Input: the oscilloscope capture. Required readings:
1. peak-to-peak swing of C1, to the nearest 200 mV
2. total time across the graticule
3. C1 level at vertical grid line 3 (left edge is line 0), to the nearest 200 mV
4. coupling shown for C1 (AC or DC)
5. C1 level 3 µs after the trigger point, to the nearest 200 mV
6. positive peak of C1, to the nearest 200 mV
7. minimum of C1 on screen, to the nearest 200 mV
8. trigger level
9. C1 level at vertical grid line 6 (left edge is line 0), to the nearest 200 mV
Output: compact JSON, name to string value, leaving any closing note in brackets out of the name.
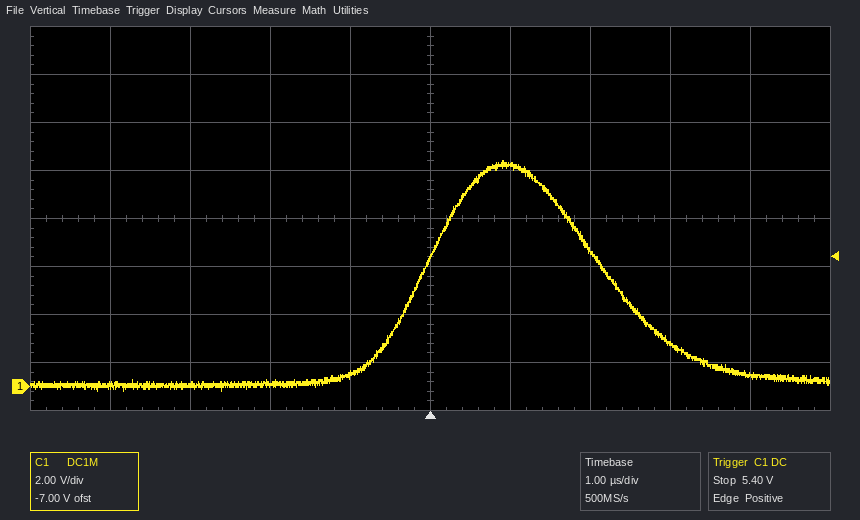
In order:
{"peak-to-peak swing of C1, to the nearest 200 mV": "9.6 V", "total time across the graticule": "10 µs", "C1 level at vertical grid line 3 (left edge is line 0), to the nearest 200 mV": "200 mV", "coupling shown for C1": "DC", "C1 level 3 µs after the trigger point, to the nearest 200 mV": "1.8 V", "positive peak of C1, to the nearest 200 mV": "9.4 V", "minimum of C1 on screen, to the nearest 200 mV": "-200 mV", "trigger level": "5.40 V", "C1 level at vertical grid line 6 (left edge is line 0), to the nearest 200 mV": "9.2 V"}
